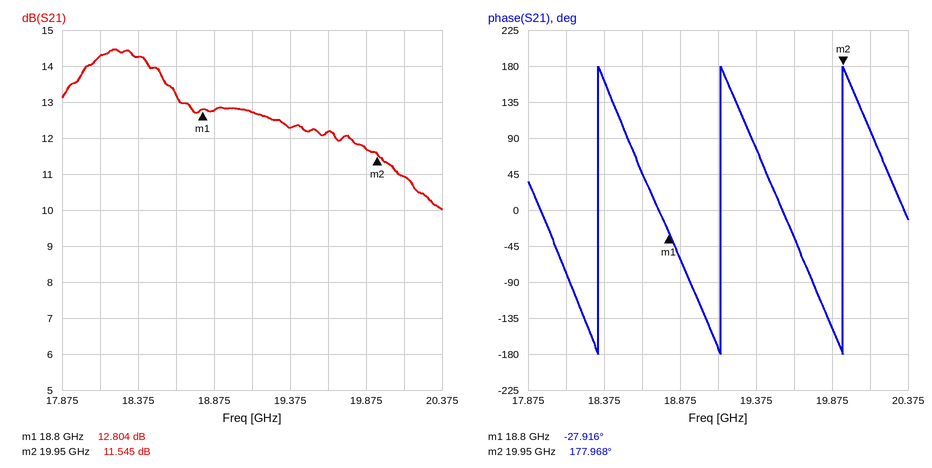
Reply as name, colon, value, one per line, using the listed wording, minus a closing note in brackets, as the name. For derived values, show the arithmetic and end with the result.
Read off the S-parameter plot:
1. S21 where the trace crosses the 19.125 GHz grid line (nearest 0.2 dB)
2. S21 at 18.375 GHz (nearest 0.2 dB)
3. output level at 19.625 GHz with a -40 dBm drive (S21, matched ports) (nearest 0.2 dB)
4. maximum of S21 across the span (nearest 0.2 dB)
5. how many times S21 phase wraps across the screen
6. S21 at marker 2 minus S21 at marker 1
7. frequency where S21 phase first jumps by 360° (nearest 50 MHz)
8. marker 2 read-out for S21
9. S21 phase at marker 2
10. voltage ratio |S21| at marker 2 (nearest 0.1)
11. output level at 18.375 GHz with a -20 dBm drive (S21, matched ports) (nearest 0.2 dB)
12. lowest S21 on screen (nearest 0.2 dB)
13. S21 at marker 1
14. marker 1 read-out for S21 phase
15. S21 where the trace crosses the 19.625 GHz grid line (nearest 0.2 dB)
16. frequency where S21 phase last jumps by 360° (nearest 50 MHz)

S21 where the trace crosses the 19.125 GHz grid line: 12.8 dB
S21 at 18.375 GHz: 14.2 dB
output level at 19.625 GHz with a -40 dBm drive (S21, matched ports): -40 dBm + (12.2 dB) = -27.8 dBm
maximum of S21 across the span: 14.4 dB
how many times S21 phase wraps across the screen: 3
S21 at marker 2 minus S21 at marker 1: 11.545 − (12.804) = -1.259 dB
frequency where S21 phase first jumps by 360°: 18.35 GHz
marker 2 read-out for S21: 11.545 dB
S21 phase at marker 2: 177.968°
voltage ratio |S21| at marker 2: 10^(11.545/20) ≈ 3.8
output level at 18.375 GHz with a -20 dBm drive (S21, matched ports): -20 dBm + (14.2 dB) = -5.8 dBm
lowest S21 on screen: 10.0 dB
S21 at marker 1: 12.804 dB
marker 1 read-out for S21 phase: -27.916°
S21 where the trace crosses the 19.625 GHz grid line: 12.2 dB
frequency where S21 phase last jumps by 360°: 19.95 GHz
